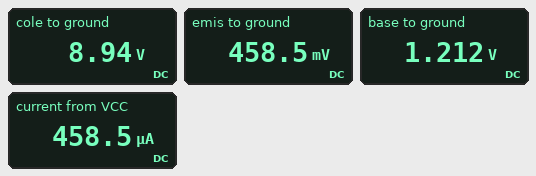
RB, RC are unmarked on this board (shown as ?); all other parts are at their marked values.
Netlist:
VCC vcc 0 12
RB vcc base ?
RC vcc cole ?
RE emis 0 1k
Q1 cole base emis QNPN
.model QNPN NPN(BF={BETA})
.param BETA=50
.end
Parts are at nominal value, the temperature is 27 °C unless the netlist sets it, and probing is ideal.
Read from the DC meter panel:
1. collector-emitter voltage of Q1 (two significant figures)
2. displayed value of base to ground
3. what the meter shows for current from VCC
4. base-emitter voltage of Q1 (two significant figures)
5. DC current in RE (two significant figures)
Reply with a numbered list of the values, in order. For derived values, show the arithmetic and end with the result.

1. 8.94 V - 458.5 mV = 8.5 V
2. 1.212 V
3. 458.5 µA
4. 1.212 V - 458.5 mV = 750 mV
5. (458.5 mV) / 1 kΩ = 460 µA
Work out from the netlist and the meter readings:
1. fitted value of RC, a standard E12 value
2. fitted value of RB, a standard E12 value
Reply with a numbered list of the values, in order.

1. 6.8 kΩ
2. 1.2 MΩ
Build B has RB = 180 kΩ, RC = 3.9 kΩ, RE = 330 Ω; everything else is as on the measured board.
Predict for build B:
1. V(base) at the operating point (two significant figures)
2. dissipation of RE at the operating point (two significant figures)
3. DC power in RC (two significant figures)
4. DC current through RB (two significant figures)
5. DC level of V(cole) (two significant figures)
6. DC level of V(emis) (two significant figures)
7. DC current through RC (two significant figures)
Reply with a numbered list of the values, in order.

1. 1.7 V
2. 2.7 mW
3. 30 mW
4. 57 µA
5. 1.1 V
6. 940 mV
7. 2.8 mA
